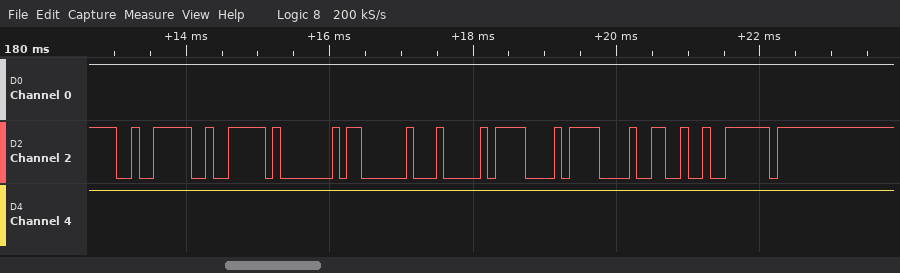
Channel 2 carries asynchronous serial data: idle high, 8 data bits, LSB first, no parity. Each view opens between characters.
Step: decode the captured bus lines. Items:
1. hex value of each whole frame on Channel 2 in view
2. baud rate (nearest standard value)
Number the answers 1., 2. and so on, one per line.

1. F2, F2, 01, 03, 04, 0F, 0F, 26, 7E
2. 9600 baud
